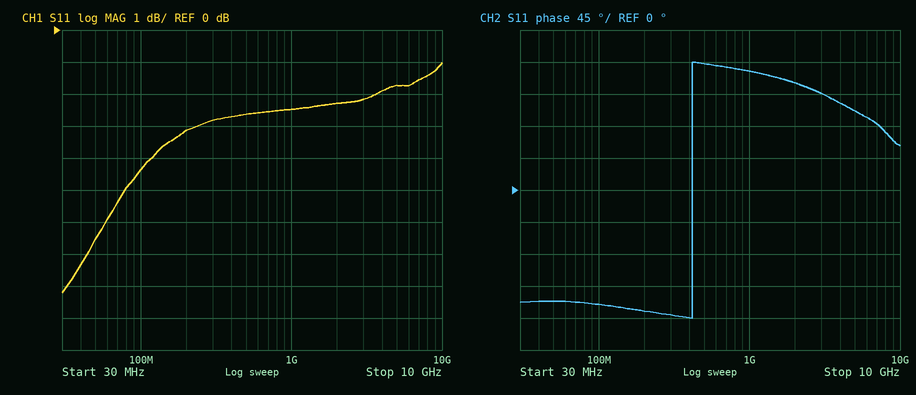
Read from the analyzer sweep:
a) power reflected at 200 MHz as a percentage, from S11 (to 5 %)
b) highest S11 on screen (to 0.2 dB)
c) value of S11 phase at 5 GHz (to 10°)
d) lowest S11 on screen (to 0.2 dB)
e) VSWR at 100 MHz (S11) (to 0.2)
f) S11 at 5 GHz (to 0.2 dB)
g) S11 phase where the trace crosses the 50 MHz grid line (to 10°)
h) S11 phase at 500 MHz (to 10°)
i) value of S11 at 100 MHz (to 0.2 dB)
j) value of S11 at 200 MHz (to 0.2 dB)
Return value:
50 %
-1.0 dB
110°
-8.2 dB
4.0
-1.8 dB
-160°
180°
-4.4 dB
-3.2 dB
